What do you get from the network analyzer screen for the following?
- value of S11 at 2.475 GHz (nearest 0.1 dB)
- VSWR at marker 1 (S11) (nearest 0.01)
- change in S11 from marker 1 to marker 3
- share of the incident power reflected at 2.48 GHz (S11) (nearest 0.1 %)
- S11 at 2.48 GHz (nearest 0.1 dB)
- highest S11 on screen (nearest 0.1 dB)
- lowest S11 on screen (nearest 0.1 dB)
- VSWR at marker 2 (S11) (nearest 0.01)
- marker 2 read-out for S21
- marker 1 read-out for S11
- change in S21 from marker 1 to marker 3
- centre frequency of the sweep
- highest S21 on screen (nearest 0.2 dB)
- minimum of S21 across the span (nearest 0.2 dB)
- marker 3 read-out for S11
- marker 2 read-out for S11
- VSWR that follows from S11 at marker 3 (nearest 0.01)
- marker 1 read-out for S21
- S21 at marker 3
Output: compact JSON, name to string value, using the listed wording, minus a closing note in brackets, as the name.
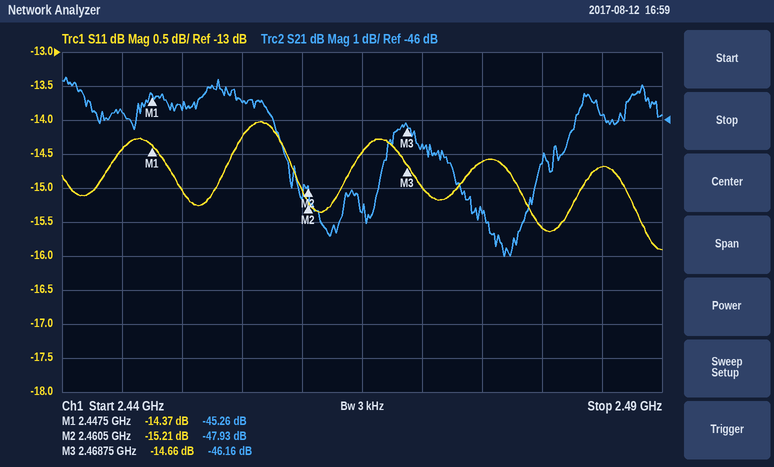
{"value of S11 at 2.475 GHz": "-14.6 dB", "VSWR at marker 1 (S11)": "1.47", "change in S11 from marker 1 to marker 3": "-0.29 dB", "share of the incident power reflected at 2.48 GHz (S11)": "2.8 %", "S11 at 2.48 GHz": "-15.6 dB", "highest S11 on screen": "-14.0 dB", "lowest S11 on screen": "-15.9 dB", "VSWR at marker 2 (S11)": "1.42", "marker 2 read-out for S21": "-47.93 dB", "marker 1 read-out for S11": "-14.37 dB", "change in S21 from marker 1 to marker 3": "-0.90 dB", "centre frequency of the sweep": "2.465 GHz", "highest S21 on screen": "-44.8 dB", "minimum of S21 across the span": "-50.0 dB", "marker 3 read-out for S11": "-14.66 dB", "marker 2 read-out for S11": "-15.21 dB", "VSWR that follows from S11 at marker 3": "1.45", "marker 1 read-out for S21": "-45.26 dB", "S21 at marker 3": "-46.16 dB"}
